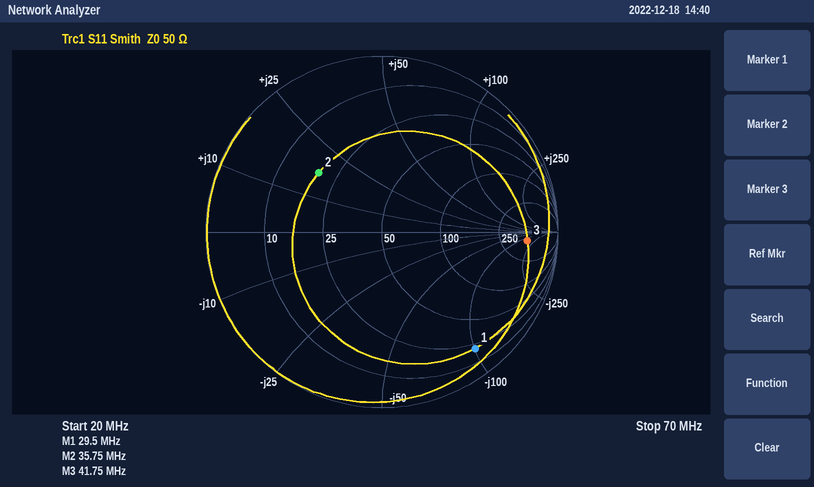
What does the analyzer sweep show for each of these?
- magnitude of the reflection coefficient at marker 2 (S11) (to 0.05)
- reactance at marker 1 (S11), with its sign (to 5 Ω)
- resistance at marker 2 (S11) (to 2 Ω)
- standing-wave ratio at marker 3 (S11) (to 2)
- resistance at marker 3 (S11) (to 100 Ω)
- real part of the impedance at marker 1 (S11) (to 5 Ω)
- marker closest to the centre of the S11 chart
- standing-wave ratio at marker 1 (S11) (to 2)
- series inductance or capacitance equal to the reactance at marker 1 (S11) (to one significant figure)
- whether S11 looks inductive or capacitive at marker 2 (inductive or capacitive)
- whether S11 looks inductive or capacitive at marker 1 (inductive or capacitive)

0.50
-100 Ω
20 Ω
10
500 Ω
20 Ω
marker 2
12
50 pF
inductive
capacitive
